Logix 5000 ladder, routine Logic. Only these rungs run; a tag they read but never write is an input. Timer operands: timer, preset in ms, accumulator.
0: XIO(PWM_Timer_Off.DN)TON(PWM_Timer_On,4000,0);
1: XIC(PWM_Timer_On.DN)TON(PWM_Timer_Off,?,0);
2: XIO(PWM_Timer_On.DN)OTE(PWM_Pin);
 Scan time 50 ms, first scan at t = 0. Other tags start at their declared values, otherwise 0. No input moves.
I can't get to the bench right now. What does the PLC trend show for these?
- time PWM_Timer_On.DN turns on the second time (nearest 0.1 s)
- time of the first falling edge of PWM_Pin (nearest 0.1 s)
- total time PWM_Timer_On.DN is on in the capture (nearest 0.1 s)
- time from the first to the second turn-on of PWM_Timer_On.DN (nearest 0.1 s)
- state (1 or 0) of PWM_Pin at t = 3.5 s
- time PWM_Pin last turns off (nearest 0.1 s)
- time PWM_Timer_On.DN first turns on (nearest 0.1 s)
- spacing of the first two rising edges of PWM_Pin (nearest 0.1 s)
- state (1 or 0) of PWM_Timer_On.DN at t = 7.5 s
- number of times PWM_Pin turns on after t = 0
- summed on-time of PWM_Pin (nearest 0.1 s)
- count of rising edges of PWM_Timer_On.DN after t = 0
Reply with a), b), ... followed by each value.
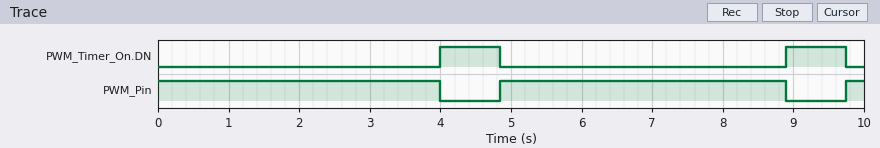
a) 8.9 s
b) 4.0 s
c) 1.7 s
d) 4.9 s
e) 1
f) 8.9 s
g) 4.0 s
h) 4.9 s
i) 0
j) 2
k) 8.3 s
l) 2
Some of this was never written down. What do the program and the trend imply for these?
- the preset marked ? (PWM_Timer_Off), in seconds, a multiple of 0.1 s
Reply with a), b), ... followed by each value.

a) 0.8 s
